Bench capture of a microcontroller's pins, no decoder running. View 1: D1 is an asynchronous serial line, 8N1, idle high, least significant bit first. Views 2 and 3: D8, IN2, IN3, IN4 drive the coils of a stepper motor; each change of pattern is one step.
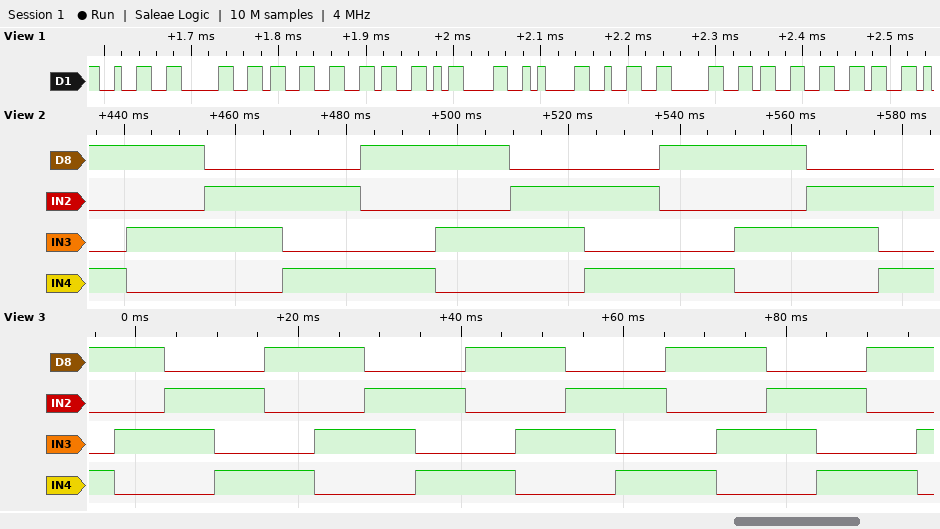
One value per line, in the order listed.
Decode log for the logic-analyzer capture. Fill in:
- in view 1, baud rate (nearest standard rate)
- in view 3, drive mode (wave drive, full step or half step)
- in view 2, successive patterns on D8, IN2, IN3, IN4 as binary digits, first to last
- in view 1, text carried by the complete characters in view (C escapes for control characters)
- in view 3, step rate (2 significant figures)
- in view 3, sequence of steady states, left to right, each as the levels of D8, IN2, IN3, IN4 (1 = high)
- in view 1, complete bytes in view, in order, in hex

115200 baud
full step
1001 1010 0110 0101 1001 1010 0110 0101 1001 1010 0110 0101
"2036\r\n2036"
160 steps/s
1001 1010 0110 0101 1001 1010 0110 0101 1001 1010 0110 0101 1001 1010 0110 0101 1001 1010
32 30 33 36 0D 0A 32 30 33 36
